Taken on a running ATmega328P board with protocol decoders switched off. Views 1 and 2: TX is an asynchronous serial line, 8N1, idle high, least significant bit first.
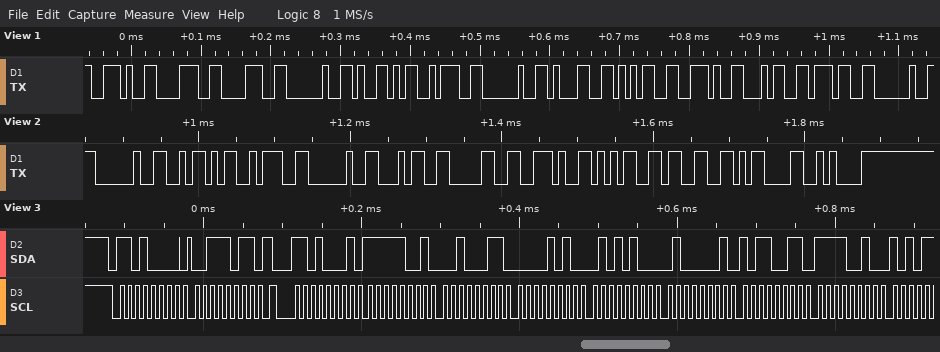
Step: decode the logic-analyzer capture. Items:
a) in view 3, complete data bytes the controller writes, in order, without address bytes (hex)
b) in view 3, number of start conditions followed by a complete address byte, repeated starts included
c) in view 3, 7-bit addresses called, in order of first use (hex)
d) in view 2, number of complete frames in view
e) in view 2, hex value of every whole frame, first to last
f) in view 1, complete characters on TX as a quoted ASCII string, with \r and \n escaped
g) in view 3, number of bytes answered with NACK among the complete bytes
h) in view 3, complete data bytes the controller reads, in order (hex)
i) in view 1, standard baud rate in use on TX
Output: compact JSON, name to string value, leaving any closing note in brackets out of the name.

{"in view 3, complete data bytes the controller writes, in order, without address bytes": "3B", "in view 3, number of start conditions followed by a complete address byte, repeated starts included": "2", "in view 3, 7-bit addresses called, in order of first use": "0x68", "in view 2, number of complete frames in view": "11", "in view 2, hex value of every whole frame, first to last": "0x20 0x5A 0x3A 0x20 0x34 0x30 0x2E 0x35 0x33 0x0D 0x0A", "in view 1, complete characters on TX as a quoted ASCII string, with \\r and \\n escaped": "\".88 Y: 15.47 \"", "in view 3, number of bytes answered with NACK among the complete bytes": "0", "in view 3, complete data bytes the controller reads, in order": "F9 23 0A 54 41 B3 F2", "in view 1, standard baud rate in use on TX": "115200 baud"}
